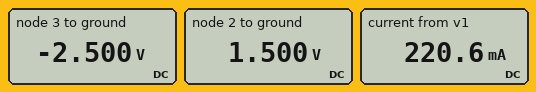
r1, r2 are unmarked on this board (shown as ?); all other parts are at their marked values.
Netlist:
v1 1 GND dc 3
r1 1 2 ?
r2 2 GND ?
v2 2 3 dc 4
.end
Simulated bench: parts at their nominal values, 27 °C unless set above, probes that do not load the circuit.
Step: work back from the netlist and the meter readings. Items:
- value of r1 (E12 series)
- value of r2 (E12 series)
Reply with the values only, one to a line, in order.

6.8 Ω
6.8 Ω
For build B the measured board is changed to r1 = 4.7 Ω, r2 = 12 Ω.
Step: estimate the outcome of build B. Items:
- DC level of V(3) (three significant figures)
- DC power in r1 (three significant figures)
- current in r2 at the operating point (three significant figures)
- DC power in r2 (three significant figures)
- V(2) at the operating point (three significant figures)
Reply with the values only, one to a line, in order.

-1.84 V
152 mW
180 mA
387 mW
2.16 V
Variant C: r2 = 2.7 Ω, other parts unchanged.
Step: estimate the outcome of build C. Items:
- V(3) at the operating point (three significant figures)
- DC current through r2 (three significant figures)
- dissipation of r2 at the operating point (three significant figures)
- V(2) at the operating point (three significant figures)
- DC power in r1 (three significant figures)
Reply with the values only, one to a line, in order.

-3.15 V
316 mA
269 mW
853 mV
678 mW
